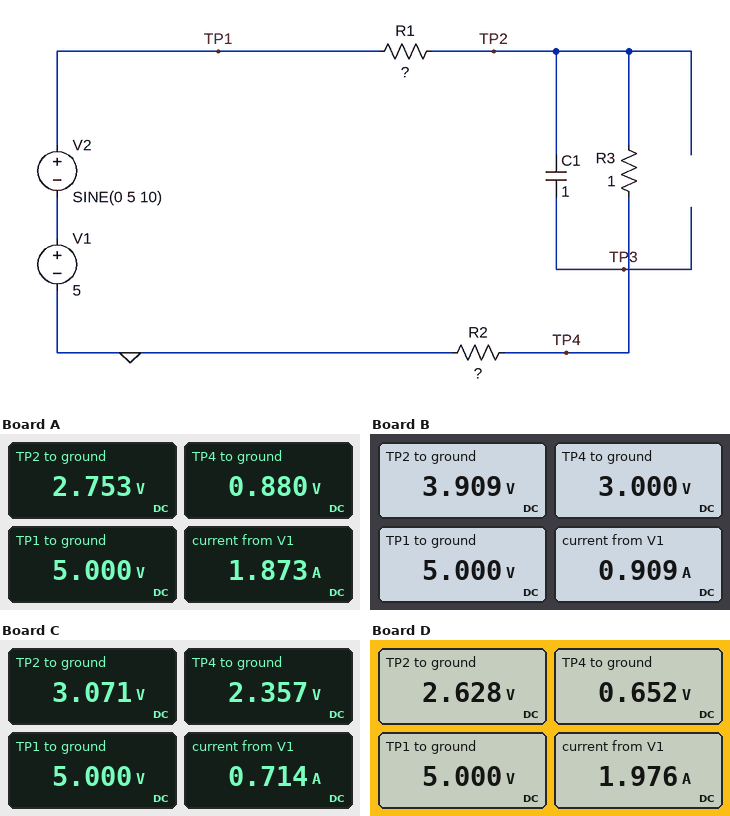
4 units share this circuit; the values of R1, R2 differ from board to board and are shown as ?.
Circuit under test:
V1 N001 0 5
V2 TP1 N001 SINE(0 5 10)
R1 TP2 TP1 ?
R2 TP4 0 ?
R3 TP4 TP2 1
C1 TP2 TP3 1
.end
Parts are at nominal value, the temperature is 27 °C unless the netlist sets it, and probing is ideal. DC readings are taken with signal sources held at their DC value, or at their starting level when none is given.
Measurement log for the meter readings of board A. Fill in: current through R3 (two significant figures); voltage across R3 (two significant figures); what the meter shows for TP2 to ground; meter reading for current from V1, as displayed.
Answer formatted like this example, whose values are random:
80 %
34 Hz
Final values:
1.9 A
1.9 V
2.753 V
1.873 A
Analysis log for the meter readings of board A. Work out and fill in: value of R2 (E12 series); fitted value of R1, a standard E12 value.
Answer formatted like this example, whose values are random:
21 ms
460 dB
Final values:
0.47 Ω
1.2 Ω
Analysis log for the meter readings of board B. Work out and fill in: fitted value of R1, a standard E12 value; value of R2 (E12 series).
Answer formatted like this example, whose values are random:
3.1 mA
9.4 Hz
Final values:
1.2 Ω
3.3 Ω
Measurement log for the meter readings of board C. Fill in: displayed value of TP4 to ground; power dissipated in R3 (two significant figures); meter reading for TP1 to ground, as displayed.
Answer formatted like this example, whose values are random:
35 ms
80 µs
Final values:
2.357 V
510 mW
5.000 V
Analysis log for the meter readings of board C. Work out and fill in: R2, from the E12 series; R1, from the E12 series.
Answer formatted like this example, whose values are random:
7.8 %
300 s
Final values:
3.3 Ω
2.7 Ω
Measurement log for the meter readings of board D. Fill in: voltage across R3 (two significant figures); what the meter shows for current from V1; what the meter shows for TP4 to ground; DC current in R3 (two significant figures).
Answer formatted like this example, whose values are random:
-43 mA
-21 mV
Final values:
2.0 V
1.976 A
0.652 V
2.0 A
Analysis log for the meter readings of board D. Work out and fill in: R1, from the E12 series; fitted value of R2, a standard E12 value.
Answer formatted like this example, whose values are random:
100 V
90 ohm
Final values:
1.2 Ω
0.33 Ω
